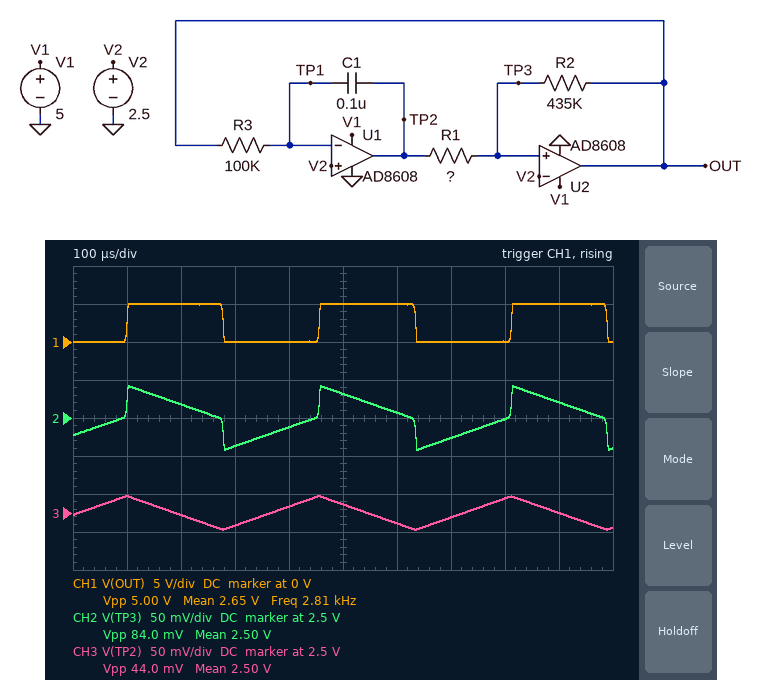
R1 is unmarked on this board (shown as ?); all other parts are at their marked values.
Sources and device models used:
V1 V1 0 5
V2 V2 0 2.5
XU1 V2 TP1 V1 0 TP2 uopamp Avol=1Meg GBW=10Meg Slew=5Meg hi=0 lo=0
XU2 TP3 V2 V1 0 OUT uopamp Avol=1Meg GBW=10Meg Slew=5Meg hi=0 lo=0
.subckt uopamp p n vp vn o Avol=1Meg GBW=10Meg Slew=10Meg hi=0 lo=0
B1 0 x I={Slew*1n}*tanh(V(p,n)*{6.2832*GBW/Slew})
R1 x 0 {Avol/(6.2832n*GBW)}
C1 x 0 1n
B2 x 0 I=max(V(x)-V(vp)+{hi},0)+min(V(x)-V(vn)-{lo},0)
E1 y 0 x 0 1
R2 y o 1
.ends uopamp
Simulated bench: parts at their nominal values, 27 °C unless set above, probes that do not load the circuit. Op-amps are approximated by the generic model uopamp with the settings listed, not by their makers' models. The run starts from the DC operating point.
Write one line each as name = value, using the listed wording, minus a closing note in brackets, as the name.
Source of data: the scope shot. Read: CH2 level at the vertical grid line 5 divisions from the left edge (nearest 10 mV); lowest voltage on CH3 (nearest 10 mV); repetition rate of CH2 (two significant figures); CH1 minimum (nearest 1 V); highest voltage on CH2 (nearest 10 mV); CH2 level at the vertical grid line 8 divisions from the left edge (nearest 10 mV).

CH2 level at the vertical grid line 5 divisions from the left edge = 2.53 V
lowest voltage on CH3 = 2.48 V
repetition rate of CH2 = 2.8 kHz
CH1 minimum = 0 V
highest voltage on CH2 = 2.54 V
CH2 level at the vertical grid line 8 divisions from the left edge = 2.50 V
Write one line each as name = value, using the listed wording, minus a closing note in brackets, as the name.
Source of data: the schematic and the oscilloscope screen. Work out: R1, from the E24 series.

R1, from the E24 series = 3.6 kΩ
